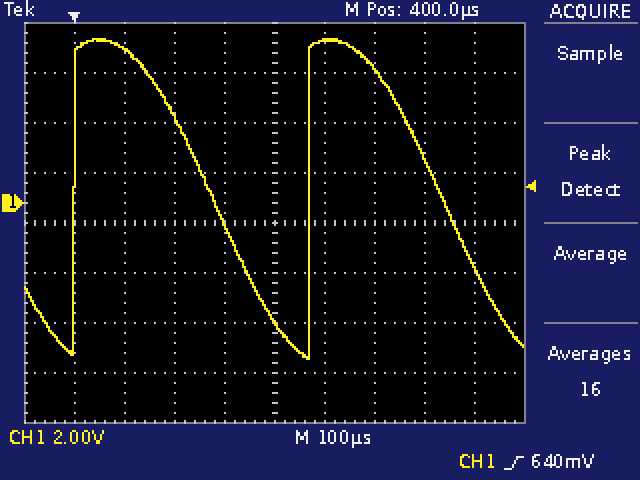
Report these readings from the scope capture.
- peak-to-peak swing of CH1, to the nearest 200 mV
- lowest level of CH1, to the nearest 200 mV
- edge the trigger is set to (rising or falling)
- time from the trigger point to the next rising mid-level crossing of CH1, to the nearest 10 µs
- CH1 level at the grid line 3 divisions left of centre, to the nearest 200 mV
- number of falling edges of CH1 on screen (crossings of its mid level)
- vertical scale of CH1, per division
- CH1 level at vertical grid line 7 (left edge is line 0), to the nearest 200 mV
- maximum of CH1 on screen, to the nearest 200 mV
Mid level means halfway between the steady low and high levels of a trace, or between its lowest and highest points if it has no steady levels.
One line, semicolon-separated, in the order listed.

12.8 V; -6.2 V; rising; 470 µs; 6.2 V; 2; 2 V; 5.4 V; 6.6 V
